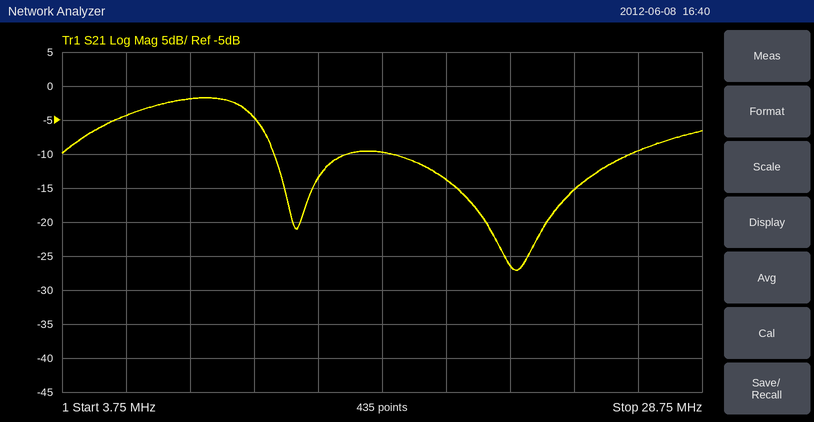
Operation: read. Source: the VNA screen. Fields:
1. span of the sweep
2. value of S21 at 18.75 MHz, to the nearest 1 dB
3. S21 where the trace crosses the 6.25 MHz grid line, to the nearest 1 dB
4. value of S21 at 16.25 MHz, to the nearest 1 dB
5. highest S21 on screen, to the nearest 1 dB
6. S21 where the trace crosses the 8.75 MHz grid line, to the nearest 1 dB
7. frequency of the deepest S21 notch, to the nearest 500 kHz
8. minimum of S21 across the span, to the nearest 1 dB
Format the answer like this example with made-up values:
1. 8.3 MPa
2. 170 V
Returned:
1. 25 MHz
2. -14 dB
3. -4 dB
4. -10 dB
5. -2 dB
6. -2 dB
7. 21.5 MHz
8. -27 dB
